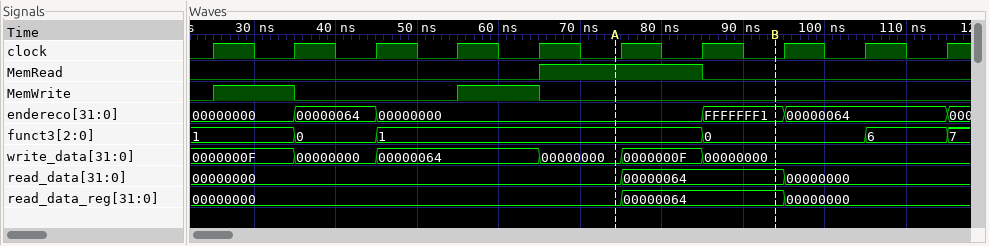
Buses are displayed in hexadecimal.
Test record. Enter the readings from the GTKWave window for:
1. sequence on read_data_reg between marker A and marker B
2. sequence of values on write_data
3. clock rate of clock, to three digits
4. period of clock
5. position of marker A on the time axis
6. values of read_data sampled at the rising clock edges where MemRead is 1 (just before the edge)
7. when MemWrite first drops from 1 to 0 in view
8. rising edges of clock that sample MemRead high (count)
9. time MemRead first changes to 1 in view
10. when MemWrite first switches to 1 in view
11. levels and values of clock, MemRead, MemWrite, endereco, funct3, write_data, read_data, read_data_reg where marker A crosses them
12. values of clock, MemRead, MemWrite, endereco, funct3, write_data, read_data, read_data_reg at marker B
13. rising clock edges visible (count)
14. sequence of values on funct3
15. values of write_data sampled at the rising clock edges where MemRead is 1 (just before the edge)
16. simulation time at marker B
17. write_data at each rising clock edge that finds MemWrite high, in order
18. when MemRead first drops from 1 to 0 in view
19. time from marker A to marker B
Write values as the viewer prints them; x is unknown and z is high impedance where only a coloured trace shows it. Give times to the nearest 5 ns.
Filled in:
00000000, 00000064
0000000F, 00000000, 00000064, 00000000, 0000000F, 00000000
100 MHz
10 ns
75 ns
00000000, 00000064
35 ns
2
65 ns
25 ns
clock=0, MemRead=1, MemWrite=0, endereco=00000000, funct3=1, write_data=00000000, read_data=00000000, read_data_reg=00000000
clock=0, MemRead=0, MemWrite=0, endereco=FFFFFFF1, funct3=0, write_data=00000000, read_data=00000064, read_data_reg=00000064
10
1, 0, 1, 0, 6, 7
00000000, 0000000F
95 ns
0000000F, 00000064
85 ns
20 ns
